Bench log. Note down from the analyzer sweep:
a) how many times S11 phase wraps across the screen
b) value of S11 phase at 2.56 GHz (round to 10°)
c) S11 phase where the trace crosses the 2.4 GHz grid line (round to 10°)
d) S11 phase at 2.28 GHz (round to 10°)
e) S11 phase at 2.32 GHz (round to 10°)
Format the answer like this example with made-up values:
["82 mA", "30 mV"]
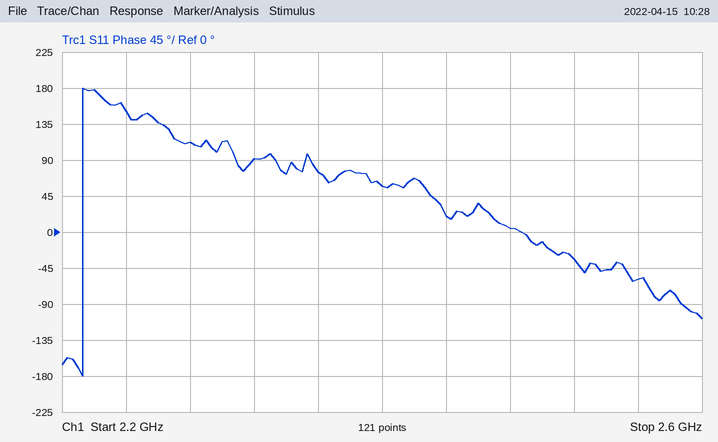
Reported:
["1", "-60°", "60°", "110°", "90°"]
